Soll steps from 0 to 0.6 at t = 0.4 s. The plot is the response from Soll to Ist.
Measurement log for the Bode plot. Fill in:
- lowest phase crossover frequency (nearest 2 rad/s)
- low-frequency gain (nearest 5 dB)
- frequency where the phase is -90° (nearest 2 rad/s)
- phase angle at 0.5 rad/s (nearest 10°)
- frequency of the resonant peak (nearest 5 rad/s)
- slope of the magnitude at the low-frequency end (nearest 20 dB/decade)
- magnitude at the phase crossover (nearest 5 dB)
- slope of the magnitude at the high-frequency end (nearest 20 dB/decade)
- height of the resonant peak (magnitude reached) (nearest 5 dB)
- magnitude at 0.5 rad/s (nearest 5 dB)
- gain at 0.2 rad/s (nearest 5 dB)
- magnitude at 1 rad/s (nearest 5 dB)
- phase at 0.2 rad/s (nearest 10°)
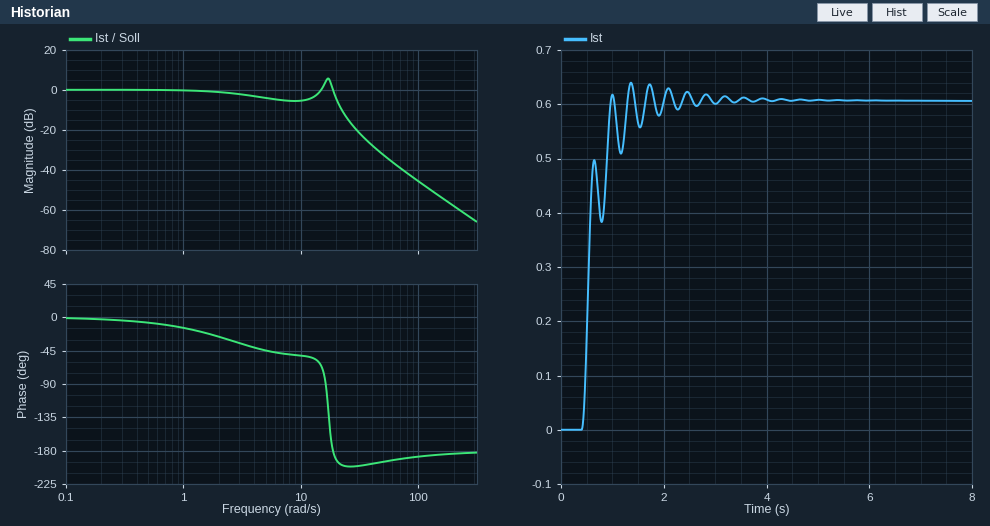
18 rad/s
0 dB
16 rad/s
-10°
15 rad/s
0 dB/decade
0 dB
-40 dB/decade
5 dB
0 dB
0 dB
0 dB
0°
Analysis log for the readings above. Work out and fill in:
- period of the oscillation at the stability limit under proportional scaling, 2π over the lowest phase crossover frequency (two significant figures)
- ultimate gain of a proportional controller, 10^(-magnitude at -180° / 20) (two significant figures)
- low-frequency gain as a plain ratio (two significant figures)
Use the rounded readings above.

0.35 s
1.0
1.0
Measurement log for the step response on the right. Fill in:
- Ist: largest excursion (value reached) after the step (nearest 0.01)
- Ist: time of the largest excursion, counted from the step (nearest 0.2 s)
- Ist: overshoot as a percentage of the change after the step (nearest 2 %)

0.64
1.0 s
6 %
